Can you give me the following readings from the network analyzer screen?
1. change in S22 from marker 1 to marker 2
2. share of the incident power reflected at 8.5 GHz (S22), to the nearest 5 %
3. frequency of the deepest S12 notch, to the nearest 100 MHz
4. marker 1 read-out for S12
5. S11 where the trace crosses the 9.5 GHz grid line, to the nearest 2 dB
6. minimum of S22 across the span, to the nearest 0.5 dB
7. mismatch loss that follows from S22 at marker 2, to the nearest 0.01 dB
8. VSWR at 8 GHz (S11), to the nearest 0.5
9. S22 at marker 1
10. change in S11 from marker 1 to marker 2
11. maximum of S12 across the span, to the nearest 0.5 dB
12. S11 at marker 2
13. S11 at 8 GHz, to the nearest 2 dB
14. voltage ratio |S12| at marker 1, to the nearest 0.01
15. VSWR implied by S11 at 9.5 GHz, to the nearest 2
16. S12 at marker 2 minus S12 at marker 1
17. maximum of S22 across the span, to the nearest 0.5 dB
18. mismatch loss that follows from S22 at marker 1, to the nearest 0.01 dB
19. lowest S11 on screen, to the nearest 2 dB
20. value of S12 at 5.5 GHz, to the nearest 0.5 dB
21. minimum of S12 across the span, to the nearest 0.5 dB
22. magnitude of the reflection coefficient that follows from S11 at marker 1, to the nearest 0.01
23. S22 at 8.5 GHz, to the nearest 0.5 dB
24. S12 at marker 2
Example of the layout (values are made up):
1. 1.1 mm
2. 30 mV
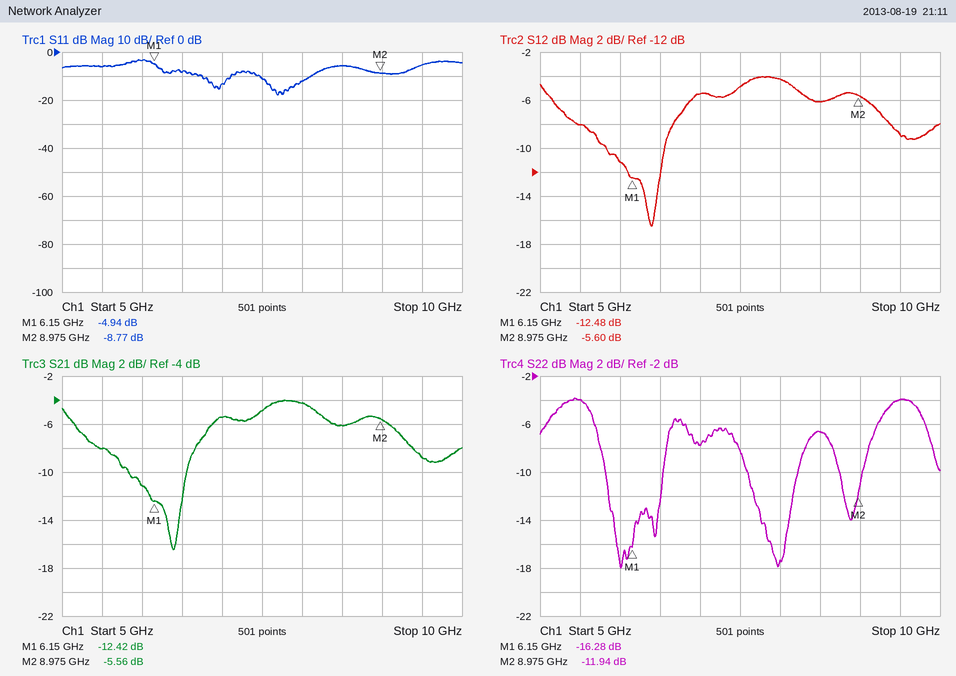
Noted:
1. 4.34 dB
2. 20 %
3. 6.4 GHz
4. -12.48 dB
5. -6 dB
6. -18.0 dB
7. 0.29 dB
8. 1.5
9. -16.28 dB
10. -3.83 dB
11. -4.0 dB
12. -8.77 dB
13. -12 dB
14. 0.24
15. 4
16. 6.88 dB
17. -4.0 dB
18. 0.10 dB
19. -18 dB
20. -8.0 dB
21. -16.5 dB
22. 0.57
23. -6.5 dB
24. -5.60 dB
